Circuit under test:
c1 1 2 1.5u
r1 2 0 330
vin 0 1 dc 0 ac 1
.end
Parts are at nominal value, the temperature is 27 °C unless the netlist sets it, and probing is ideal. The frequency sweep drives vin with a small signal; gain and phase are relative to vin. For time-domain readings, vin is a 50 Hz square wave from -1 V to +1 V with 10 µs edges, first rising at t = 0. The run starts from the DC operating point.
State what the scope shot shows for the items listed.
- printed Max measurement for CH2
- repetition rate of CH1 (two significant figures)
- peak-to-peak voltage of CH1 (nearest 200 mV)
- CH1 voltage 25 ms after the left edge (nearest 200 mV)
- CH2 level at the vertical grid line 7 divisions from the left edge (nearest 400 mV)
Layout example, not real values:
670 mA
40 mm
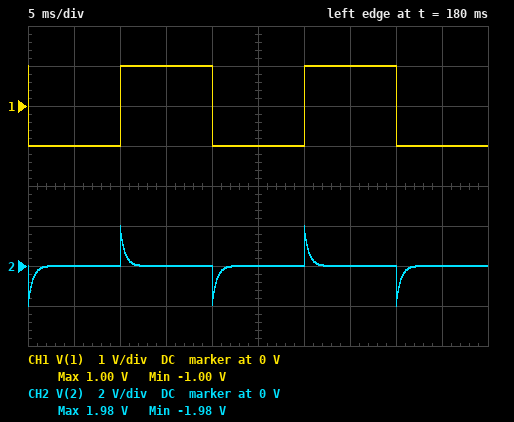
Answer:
1.98 V
50 Hz
2.0 V
-1.0 V
0 V
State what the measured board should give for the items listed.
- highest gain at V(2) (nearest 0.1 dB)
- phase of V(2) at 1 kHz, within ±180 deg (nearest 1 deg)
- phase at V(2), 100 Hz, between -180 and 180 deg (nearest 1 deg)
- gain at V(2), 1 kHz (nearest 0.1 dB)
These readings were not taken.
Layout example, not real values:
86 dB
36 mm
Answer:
0 dB
-162 deg
-107 deg
-0.4 dB
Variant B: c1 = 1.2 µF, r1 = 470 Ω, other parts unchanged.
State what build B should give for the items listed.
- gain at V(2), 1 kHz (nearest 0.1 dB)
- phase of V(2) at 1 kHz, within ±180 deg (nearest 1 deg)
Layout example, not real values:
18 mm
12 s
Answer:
-0.3 dB
-164 deg
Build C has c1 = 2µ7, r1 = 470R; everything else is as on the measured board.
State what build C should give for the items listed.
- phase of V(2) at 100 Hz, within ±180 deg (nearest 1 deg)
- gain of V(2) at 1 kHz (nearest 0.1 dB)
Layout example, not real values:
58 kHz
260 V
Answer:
-129 deg
-0.1 dB
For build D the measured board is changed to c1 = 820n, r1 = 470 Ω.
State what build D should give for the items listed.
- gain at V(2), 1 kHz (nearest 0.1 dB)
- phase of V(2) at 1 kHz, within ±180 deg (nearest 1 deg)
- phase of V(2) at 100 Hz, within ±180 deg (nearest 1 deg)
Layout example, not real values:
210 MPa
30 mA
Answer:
-0.7 dB
-158 deg
-104 deg
